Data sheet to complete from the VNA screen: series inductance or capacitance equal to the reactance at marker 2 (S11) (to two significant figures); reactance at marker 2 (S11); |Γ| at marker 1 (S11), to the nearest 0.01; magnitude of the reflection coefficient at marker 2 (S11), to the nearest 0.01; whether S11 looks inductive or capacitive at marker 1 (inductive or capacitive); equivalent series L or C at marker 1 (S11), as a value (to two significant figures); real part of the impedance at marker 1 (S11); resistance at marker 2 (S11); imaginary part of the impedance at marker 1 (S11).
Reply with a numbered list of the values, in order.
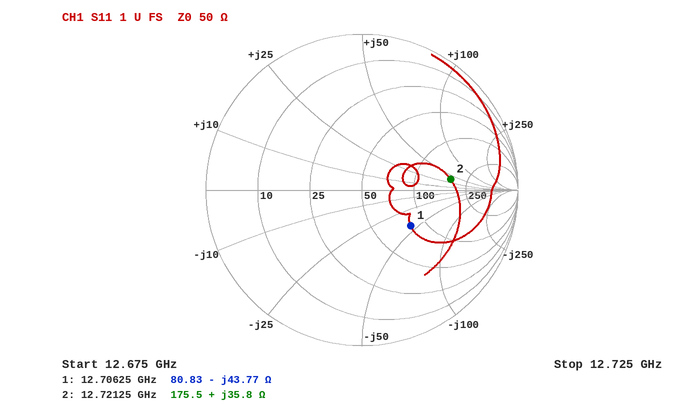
1. 450 pH
2. +35.8 Ω
3. 0.39
4. 0.57
5. capacitive
6. 290 fF
7. 80.83 Ω
8. 175.5 Ω
9. -43.77 Ω
